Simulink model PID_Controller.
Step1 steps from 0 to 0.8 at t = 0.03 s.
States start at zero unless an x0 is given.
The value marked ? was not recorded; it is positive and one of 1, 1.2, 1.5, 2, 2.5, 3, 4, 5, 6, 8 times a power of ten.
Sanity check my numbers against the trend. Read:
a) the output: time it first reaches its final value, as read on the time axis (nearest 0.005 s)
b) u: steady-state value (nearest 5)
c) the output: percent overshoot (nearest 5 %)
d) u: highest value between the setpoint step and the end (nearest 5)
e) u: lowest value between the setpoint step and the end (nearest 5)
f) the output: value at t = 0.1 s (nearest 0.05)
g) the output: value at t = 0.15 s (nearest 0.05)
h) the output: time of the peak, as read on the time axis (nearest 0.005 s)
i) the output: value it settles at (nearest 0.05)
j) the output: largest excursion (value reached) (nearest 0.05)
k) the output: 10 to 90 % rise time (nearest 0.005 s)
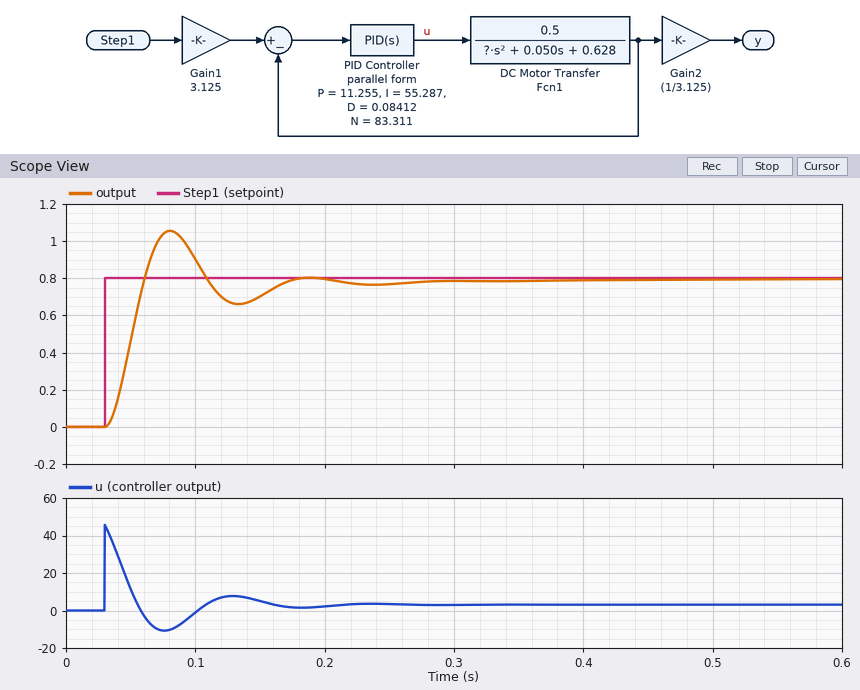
0.060 s
5
30 %
45
-10
0.90
0.70
0.080 s
0.80
1.05
0.020 s
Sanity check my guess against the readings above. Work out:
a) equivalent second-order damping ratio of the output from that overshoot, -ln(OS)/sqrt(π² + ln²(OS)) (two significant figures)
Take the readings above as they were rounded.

0.36
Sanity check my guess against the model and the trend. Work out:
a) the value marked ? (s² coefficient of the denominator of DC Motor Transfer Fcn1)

0.002
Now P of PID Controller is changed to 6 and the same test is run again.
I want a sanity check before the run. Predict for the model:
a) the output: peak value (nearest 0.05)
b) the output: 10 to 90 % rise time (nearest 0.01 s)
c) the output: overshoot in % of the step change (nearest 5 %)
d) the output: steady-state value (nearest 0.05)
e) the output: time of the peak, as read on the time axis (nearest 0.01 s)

0.95
0.03 s
20 %
0.80
0.10 s
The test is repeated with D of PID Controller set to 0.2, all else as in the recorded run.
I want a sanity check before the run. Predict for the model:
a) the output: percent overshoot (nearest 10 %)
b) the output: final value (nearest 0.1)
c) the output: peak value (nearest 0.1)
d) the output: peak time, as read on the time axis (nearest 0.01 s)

20 %
0.8
1.0
0.07 s
